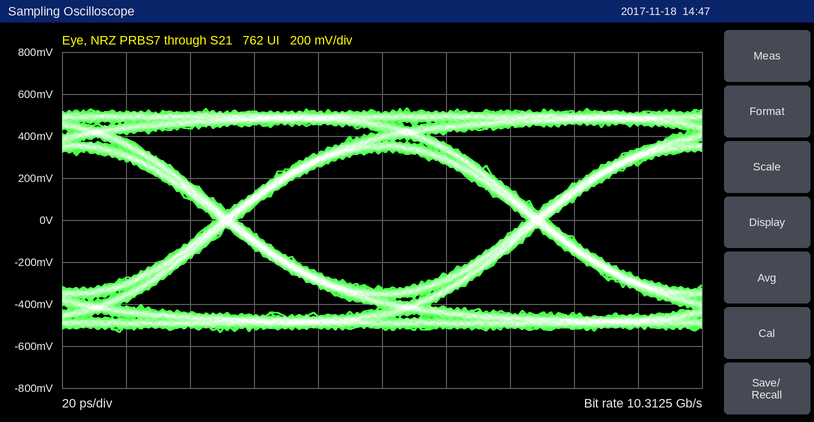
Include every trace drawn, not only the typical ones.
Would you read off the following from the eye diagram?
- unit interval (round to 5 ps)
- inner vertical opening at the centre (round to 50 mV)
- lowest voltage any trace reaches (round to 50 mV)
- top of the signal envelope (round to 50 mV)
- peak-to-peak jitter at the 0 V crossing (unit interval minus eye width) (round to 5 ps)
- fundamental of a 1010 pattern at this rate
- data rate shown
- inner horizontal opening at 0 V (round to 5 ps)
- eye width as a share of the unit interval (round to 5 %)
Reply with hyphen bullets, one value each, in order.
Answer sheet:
- 95 ps
- 650 mV
- -550 mV
- 550 mV
- 5 ps
- 5.15625 GHz
- 10.3125 Gb/s
- 90 ps
- 95 %
